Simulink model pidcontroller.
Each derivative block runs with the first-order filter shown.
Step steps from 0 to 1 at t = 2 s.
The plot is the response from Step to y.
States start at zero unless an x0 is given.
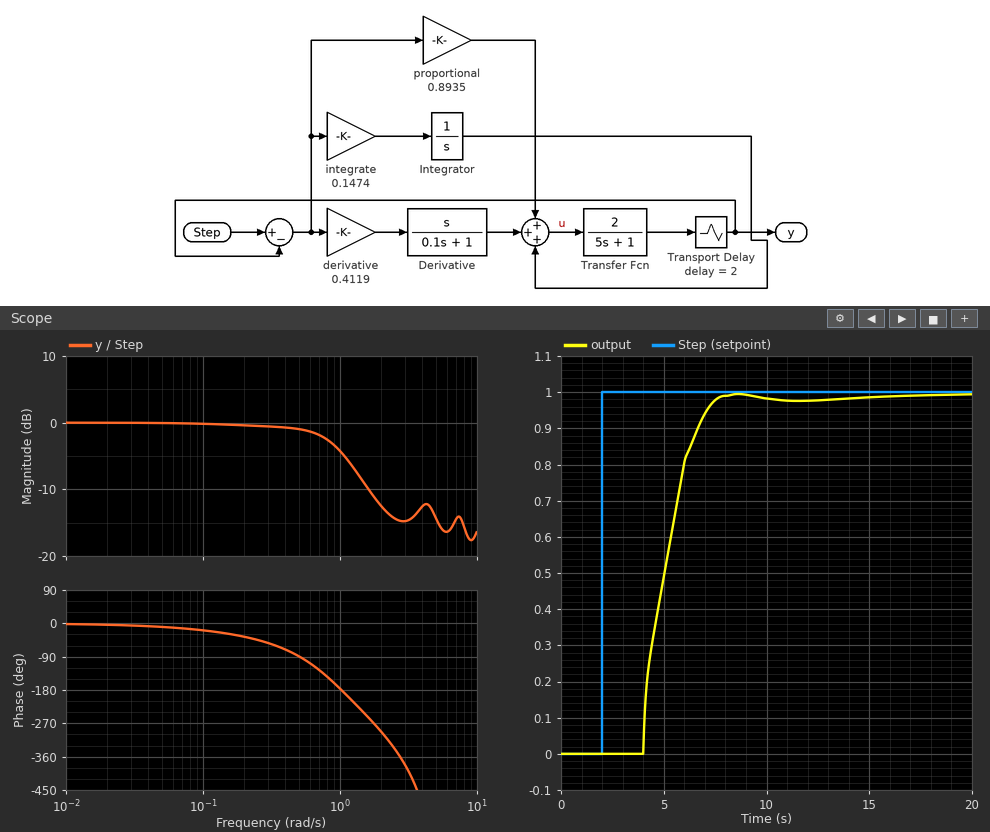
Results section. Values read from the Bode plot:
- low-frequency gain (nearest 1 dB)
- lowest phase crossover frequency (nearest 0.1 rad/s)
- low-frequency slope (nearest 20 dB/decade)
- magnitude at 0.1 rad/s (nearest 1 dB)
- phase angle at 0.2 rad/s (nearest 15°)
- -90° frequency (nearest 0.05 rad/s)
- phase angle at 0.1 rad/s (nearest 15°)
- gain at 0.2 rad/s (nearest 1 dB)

0 dB
1.0 rad/s
0 dB/decade
0 dB
-30°
0.50 rad/s
-15°
0 dB
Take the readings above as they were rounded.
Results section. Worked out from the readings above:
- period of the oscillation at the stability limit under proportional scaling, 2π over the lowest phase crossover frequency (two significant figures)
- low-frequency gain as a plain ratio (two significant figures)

6.3 s
1.0
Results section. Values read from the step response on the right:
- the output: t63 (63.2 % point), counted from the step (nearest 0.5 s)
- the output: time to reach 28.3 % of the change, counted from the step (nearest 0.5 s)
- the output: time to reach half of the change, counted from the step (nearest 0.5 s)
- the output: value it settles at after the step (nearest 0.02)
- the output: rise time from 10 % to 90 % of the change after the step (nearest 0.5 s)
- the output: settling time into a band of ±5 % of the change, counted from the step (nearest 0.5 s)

3.5 s
2.5 s
3.0 s
1.00
2.5 s
5.0 s
